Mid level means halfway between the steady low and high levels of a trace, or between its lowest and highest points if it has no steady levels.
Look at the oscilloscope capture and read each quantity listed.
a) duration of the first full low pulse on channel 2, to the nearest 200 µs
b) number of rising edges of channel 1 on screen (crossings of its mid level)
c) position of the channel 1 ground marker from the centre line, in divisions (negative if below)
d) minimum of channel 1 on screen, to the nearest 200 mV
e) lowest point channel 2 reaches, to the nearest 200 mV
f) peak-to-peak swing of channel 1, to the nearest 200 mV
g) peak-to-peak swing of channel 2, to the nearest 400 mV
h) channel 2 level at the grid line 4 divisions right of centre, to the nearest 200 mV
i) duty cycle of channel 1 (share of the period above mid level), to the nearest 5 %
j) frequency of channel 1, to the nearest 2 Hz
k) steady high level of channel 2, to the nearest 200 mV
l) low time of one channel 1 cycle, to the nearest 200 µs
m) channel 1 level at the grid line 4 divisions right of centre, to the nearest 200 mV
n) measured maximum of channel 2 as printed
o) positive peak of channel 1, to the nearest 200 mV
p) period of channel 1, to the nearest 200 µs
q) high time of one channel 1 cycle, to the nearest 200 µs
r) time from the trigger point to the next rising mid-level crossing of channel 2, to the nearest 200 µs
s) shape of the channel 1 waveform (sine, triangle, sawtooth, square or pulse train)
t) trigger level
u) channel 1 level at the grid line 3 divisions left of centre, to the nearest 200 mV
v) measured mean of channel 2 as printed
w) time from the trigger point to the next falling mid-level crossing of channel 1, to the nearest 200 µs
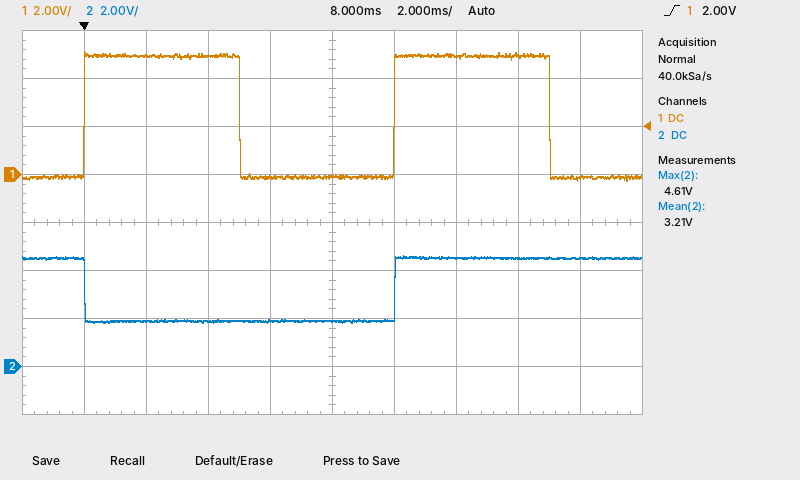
10.0 ms
2
+1.0 div
-200 mV
1.8 V
5.4 V
2.8 V
4.6 V
50 %
100 Hz
4.6 V
5.0 ms
-200 mV
4.61 V
5.2 V
10.0 ms
5.0 ms
10.0 ms
square
2.00 V
5.0 V
3.21 V
5.0 ms
